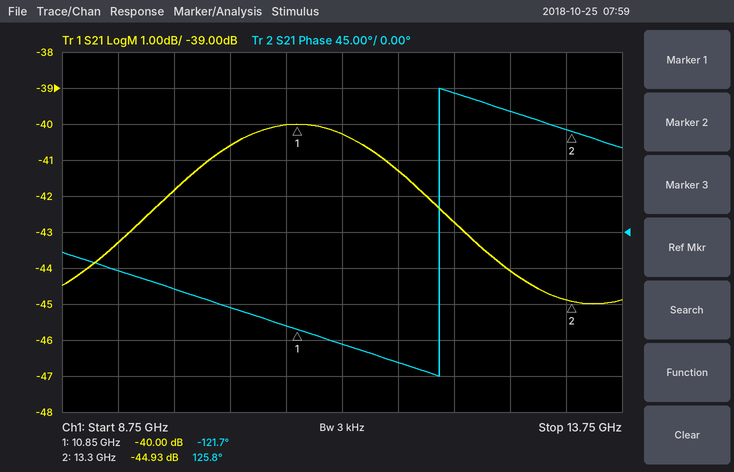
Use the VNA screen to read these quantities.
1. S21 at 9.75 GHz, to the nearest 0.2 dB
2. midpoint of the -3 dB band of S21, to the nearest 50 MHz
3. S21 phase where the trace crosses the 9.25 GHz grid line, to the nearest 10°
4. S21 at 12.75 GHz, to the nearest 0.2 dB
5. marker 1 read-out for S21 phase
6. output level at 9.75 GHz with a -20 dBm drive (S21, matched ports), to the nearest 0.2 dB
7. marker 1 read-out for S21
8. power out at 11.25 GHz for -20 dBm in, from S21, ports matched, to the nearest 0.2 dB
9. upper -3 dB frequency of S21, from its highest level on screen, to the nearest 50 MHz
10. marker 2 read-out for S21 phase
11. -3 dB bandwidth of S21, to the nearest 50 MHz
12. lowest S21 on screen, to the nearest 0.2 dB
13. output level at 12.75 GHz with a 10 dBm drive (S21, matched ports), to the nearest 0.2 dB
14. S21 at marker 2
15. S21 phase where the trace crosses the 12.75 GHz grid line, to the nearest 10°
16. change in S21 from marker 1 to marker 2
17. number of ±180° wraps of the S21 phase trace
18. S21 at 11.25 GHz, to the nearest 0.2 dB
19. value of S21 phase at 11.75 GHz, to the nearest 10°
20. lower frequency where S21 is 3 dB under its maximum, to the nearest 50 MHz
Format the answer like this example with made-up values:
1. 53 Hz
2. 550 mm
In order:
1. -41.8 dB
2. 10.85 GHz
3. -50°
4. -44.0 dB
5. -121.7°
6. -61.8 dBm
7. -40.00 dB
8. -60.2 dBm
9. 12.35 GHz
10. 125.8°
11. 3.00 GHz
12. -45.0 dB
13. -34.0 dBm
14. -44.93 dB
15. 150°
16. -4.93 dB
17. 1
18. -40.2 dB
19. -160°
20. 9.35 GHz
